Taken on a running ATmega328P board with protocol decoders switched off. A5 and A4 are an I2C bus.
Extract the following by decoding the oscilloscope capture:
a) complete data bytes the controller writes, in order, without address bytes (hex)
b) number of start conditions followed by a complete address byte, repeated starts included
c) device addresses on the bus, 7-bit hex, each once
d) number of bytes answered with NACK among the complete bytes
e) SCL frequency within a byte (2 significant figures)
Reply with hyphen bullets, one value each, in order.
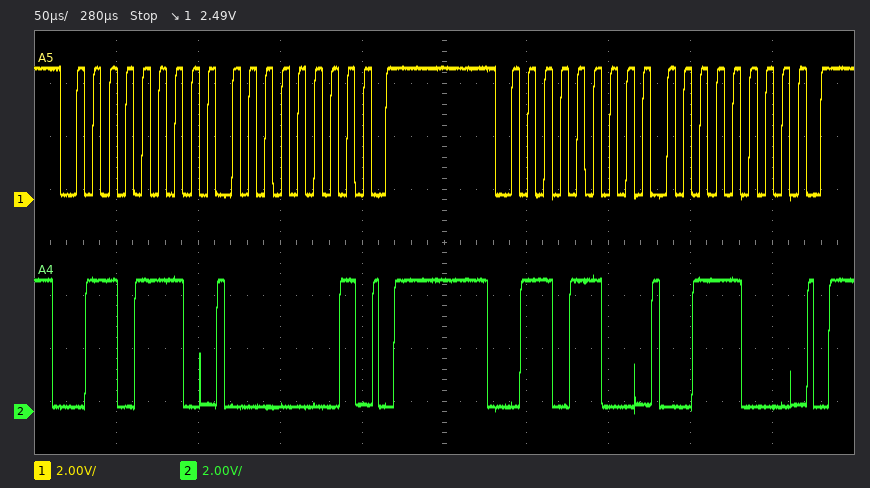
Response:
- 01 38
- 2
- 0x37 0x36
- 0
- 100 kHz
